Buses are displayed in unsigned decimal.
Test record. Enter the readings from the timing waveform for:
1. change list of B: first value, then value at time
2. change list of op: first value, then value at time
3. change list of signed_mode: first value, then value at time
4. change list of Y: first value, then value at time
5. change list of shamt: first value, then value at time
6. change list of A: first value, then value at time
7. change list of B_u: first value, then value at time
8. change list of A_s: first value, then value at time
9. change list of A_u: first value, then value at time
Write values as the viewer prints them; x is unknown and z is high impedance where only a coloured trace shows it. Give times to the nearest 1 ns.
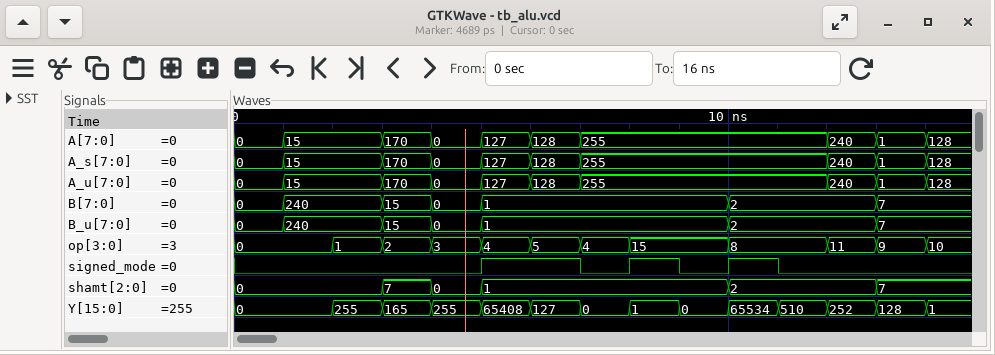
0, 240 at 1 ns, 15 at 3 ns, 0 at 4 ns, 1 at 5 ns, 2 at 10 ns, 7 at 13 ns
0, 1 at 2 ns, 2 at 3 ns, 3 at 4 ns, 4 at 5 ns, 5 at 6 ns, 4 at 7 ns, 15 at 8 ns, 8 at 10 ns, 11 at 12 ns, 9 at 13 ns, 10 at 14 ns
0, 1 at 5 ns, 0 at 7 ns, 1 at 8 ns, 0 at 9 ns, 1 at 10 ns, 0 at 11 ns
0, 255 at 2 ns, 165 at 3 ns, 255 at 4 ns, 65408 at 5 ns, 127 at 6 ns, 0 at 7 ns, 1 at 8 ns, 0 at 9 ns, 65534 at 10 ns, 510 at 11 ns, 252 at 12 ns, 128 at 13 ns, 1 at 14 ns
0, 7 at 3 ns, 0 at 4 ns, 1 at 5 ns, 2 at 10 ns, 7 at 13 ns
0, 15 at 1 ns, 170 at 3 ns, 0 at 4 ns, 127 at 5 ns, 128 at 6 ns, 255 at 7 ns, 240 at 12 ns, 1 at 13 ns, 128 at 14 ns
0, 240 at 1 ns, 15 at 3 ns, 0 at 4 ns, 1 at 5 ns, 2 at 10 ns, 7 at 13 ns
0, 15 at 1 ns, 170 at 3 ns, 0 at 4 ns, 127 at 5 ns, 128 at 6 ns, 255 at 7 ns, 240 at 12 ns, 1 at 13 ns, 128 at 14 ns
0, 15 at 1 ns, 170 at 3 ns, 0 at 4 ns, 127 at 5 ns, 128 at 6 ns, 255 at 7 ns, 240 at 12 ns, 1 at 13 ns, 128 at 14 ns
